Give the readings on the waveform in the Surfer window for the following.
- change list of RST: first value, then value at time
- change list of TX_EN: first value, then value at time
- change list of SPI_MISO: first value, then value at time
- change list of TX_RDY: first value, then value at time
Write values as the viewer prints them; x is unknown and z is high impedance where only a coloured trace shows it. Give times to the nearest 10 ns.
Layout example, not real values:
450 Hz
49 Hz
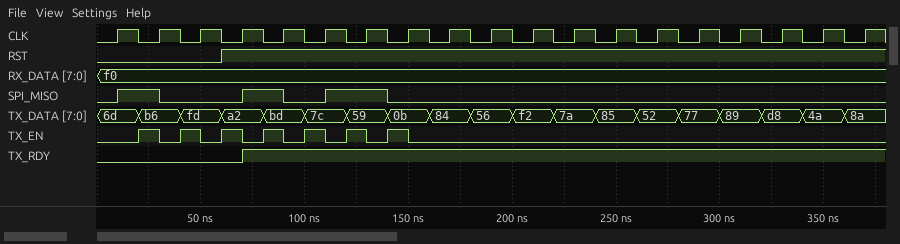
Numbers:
0, 1 at 60 ns
0, 1 at 20 ns, 0 at 30 ns, 1 at 40 ns, 0 at 50 ns, 1 at 60 ns, 0 at 70 ns, 1 at 80 ns, 0 at 90 ns, 1 at 100 ns, 0 at 110 ns, 1 at 120 ns, 0 at 130 ns, 1 at 140 ns, 0 at 150 ns
0, 1 at 10 ns, 0 at 30 ns, 1 at 70 ns, 0 at 90 ns, 1 at 110 ns, 0 at 140 ns
0, 1 at 70 ns
